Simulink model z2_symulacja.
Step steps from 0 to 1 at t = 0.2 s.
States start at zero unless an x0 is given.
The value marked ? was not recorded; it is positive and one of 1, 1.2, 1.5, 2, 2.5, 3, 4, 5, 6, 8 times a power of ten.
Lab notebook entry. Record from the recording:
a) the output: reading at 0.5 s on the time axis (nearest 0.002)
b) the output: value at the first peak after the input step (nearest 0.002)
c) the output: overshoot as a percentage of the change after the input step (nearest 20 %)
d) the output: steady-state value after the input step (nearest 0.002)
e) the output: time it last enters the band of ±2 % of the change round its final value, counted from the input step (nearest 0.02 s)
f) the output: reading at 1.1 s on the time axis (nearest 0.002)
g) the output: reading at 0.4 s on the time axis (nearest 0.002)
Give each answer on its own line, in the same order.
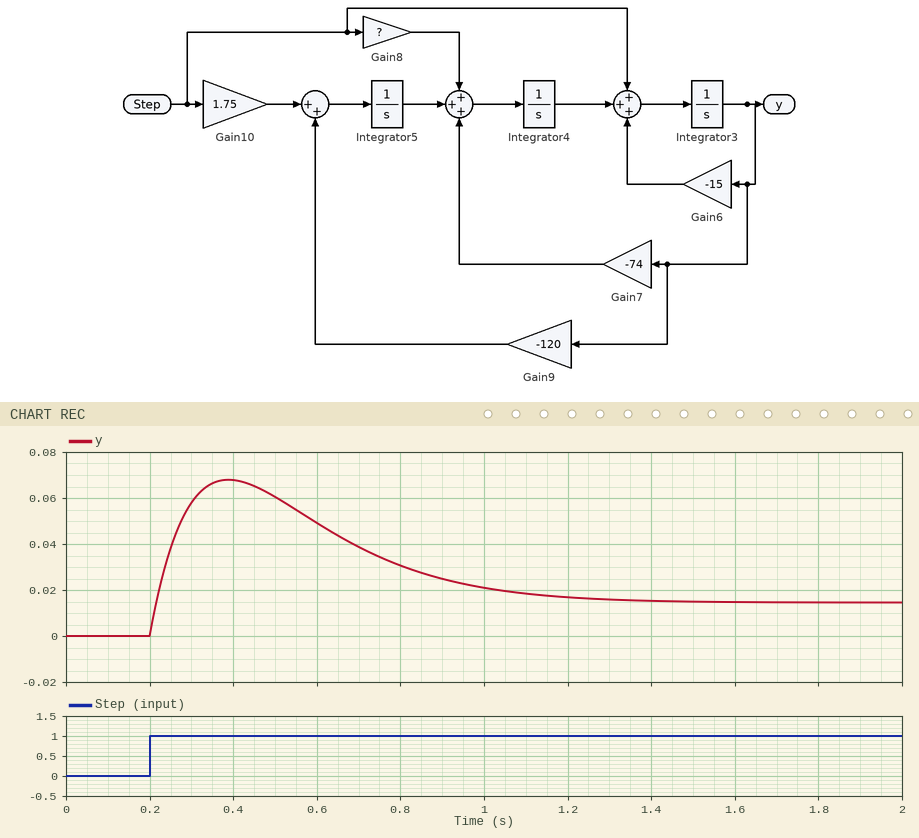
0.060
0.068
360 %
0.014
1.32 s
0.018
0.068
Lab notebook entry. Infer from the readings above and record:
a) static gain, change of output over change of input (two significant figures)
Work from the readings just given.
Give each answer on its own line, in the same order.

0.014
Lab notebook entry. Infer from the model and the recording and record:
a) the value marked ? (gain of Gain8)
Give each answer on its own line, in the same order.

4
